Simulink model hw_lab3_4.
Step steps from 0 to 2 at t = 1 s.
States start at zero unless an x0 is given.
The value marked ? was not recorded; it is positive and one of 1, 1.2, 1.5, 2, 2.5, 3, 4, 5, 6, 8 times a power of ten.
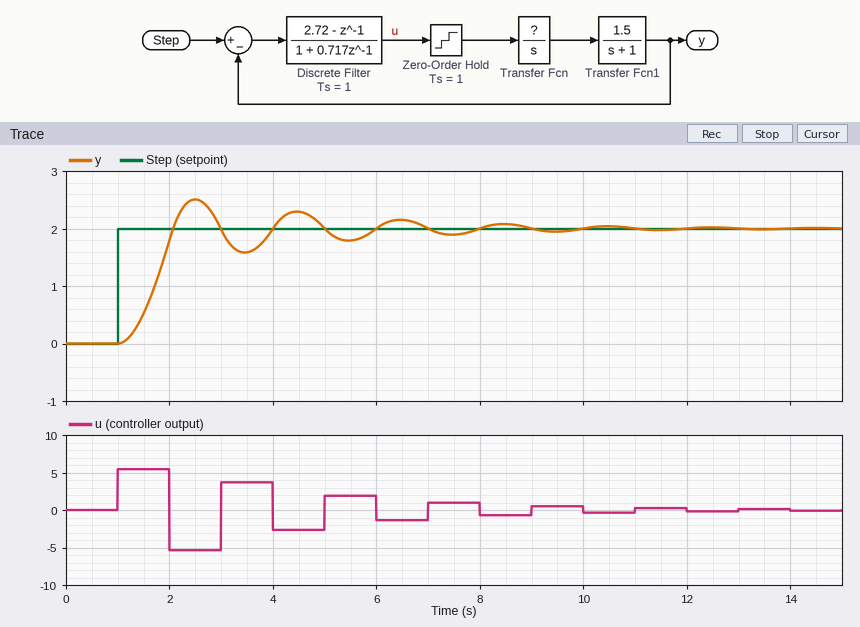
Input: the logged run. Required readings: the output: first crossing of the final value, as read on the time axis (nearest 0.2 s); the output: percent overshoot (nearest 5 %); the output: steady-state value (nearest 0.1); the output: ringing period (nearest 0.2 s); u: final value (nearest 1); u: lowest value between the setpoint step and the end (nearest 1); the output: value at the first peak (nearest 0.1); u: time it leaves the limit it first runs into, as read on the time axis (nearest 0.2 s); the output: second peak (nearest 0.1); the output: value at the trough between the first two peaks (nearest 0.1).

2.0 s
25 %
2.0
2.0 s
0
-5
2.5
2.0 s
2.3
1.6
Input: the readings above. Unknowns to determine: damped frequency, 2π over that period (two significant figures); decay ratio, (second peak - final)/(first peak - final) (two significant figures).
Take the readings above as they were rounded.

3.1 rad/s
0.60
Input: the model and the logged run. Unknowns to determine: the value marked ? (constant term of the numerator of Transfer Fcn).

0.6
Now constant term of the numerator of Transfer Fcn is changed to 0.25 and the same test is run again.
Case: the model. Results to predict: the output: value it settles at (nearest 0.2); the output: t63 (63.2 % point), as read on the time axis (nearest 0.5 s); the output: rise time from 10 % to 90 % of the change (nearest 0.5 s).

2.0
3.5 s
4.5 s
